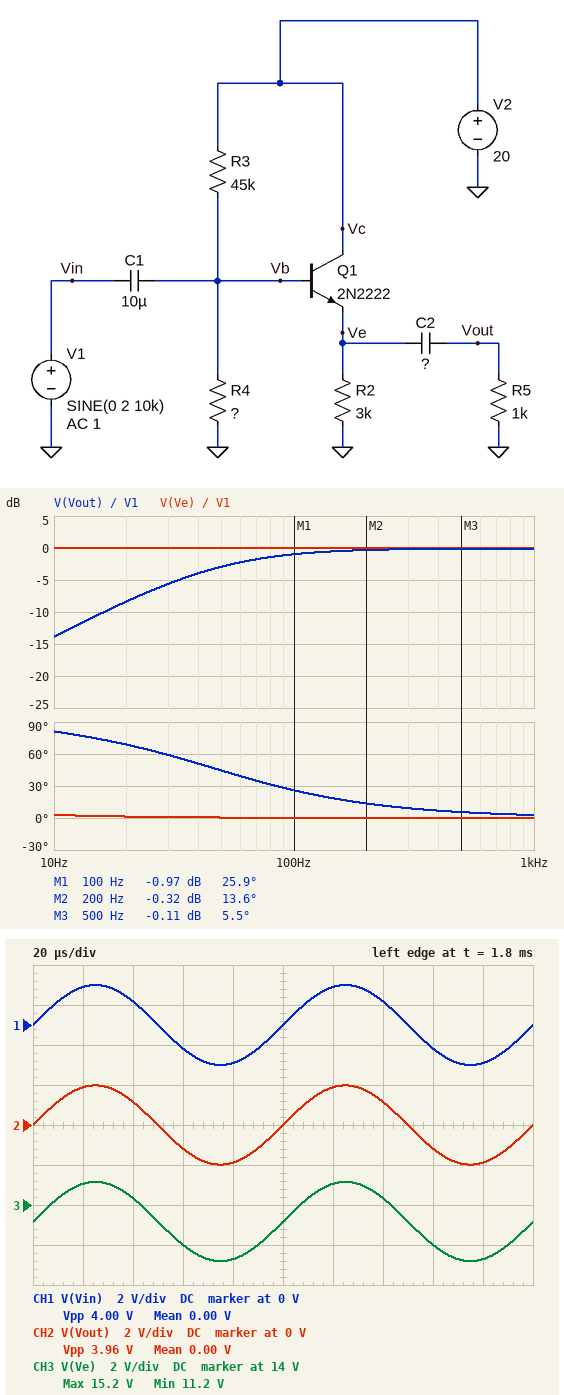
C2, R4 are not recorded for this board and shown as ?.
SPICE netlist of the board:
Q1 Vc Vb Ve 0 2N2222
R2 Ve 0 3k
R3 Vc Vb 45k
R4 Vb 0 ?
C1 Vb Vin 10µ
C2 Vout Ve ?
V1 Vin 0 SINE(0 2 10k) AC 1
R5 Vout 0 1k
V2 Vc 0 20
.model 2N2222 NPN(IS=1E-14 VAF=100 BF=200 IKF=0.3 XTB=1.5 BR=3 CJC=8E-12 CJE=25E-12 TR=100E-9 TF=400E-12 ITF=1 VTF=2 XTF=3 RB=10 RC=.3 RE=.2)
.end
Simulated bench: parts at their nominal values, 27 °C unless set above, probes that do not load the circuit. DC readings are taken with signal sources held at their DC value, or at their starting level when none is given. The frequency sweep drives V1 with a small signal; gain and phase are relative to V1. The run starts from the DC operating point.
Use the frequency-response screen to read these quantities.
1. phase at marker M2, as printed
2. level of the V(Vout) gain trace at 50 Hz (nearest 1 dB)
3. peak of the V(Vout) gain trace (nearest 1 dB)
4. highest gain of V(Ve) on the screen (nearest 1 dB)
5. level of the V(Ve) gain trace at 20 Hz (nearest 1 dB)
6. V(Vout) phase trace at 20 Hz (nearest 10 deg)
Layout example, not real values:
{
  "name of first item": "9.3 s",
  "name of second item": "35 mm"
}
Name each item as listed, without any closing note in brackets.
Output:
{
  "phase at marker M2, as printed": "13.6 deg",
  "level of the V(Vout) gain trace at 50 Hz": "-3 dB",
  "peak of the V(Vout) gain trace": "0 dB",
  "highest gain of V(Ve) on the screen": "0 dB",
  "level of the V(Ve) gain trace at 20 Hz": "0 dB",
  "V(Vout) phase trace at 20 Hz": "70 deg"
}
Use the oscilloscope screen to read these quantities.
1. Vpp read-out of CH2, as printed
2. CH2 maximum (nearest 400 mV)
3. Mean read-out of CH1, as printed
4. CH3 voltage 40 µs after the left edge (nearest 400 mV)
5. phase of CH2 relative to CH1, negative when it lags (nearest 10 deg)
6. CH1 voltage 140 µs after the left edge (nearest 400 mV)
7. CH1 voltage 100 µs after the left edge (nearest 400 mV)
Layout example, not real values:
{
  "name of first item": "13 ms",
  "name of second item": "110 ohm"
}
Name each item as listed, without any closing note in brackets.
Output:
{
  "Vpp read-out of CH2, as printed": "3.96 V",
  "CH2 maximum": "2.0 V",
  "Mean read-out of CH1, as printed": "0.00 V",
  "CH3 voltage 40 µs after the left edge": "14.4 V",
  "phase of CH2 relative to CH1, negative when it lags": "0 deg",
  "CH1 voltage 140 µs after the left edge": "1.2 V",
  "CH1 voltage 100 µs after the left edge": "0 V"
}
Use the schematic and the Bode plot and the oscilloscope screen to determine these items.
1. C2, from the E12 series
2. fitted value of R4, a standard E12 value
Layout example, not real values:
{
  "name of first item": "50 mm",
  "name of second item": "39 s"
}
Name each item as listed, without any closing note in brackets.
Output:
{
  "C2, from the E12 series": "3.3 µF",
  "fitted value of R4, a standard E12 value": "120 kΩ"
}
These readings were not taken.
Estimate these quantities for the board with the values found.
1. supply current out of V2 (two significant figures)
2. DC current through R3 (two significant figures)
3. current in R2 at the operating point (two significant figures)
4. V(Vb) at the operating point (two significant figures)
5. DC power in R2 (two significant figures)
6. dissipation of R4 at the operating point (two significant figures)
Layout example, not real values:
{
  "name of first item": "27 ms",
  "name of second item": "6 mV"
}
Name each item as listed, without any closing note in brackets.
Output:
{
  "supply current out of V2": "4.5 mA",
  "DC current through R3": "140 µA",
  "current in R2 at the operating point": "4.4 mA",
  "V(Vb) at the operating point": "14 V",
  "DC power in R2": "58 mW",
  "dissipation of R4 at the operating point": "1.6 mW"
}
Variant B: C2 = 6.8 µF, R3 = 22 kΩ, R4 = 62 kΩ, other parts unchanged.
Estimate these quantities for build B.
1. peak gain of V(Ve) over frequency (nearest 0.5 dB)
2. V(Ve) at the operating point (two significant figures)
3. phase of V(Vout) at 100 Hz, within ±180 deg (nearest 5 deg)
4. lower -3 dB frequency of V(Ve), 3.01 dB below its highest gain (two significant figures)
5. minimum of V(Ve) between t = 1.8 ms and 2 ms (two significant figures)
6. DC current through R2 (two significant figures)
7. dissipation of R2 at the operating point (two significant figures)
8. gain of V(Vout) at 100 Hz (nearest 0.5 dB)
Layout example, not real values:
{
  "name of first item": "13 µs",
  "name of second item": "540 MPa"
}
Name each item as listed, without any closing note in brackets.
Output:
{
  "peak gain of V(Ve) over frequency": "0 dB",
  "V(Ve) at the operating point": "14 V",
  "phase of V(Vout) at 100 Hz, within ±180 deg": "15 deg",
  "lower -3 dB frequency of V(Ve), 3.01 dB below its highest gain": "1.0 Hz",
  "minimum of V(Ve) between t = 1.8 ms and 2 ms": "12 V",
  "DC current through R2": "4.6 mA",
  "dissipation of R2 at the operating point": "63 mW",
  "gain of V(Vout) at 100 Hz": "-0.5 dB"
}
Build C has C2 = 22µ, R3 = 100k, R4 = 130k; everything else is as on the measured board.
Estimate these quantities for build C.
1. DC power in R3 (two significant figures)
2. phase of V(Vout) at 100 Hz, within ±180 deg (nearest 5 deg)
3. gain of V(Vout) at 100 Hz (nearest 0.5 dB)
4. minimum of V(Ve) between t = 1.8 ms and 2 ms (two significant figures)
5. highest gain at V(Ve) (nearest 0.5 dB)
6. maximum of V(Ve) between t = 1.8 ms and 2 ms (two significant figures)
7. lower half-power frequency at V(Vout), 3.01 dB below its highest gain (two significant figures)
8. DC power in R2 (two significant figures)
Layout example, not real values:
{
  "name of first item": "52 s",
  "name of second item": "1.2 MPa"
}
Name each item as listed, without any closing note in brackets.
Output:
{
  "DC power in R3": "910 µW",
  "phase of V(Vout) at 100 Hz, within ±180 deg": "5 deg",
  "gain of V(Vout) at 100 Hz": "0 dB",
  "minimum of V(Ve) between t = 1.8 ms and 2 ms": "7.8 V",
  "highest gain at V(Ve)": "0 dB",
  "maximum of V(Ve) between t = 1.8 ms and 2 ms": "12 V",
  "lower half-power frequency at V(Vout), 3.01 dB below its highest gain": "7.3 Hz",
  "DC power in R2": "32 mW"
}
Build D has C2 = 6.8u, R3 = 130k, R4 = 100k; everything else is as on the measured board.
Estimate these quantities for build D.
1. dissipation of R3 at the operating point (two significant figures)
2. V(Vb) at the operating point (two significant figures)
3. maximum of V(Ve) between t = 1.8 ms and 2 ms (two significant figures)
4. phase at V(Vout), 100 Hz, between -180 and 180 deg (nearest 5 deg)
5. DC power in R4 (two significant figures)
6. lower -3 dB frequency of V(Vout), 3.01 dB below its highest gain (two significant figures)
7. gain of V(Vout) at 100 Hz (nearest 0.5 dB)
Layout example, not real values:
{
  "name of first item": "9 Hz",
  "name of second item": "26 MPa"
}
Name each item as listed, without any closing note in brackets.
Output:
{
  "dissipation of R3 at the operating point": "1.1 mW",
  "V(Vb) at the operating point": "8.1 V",
  "maximum of V(Ve) between t = 1.8 ms and 2 ms": "9.4 V",
  "phase at V(Vout), 100 Hz, between -180 and 180 deg": "15 deg",
  "DC power in R4": "650 µW",
  "lower -3 dB frequency of V(Vout), 3.01 dB below its highest gain": "23 Hz",
  "gain of V(Vout) at 100 Hz": "-0.5 dB"
}
